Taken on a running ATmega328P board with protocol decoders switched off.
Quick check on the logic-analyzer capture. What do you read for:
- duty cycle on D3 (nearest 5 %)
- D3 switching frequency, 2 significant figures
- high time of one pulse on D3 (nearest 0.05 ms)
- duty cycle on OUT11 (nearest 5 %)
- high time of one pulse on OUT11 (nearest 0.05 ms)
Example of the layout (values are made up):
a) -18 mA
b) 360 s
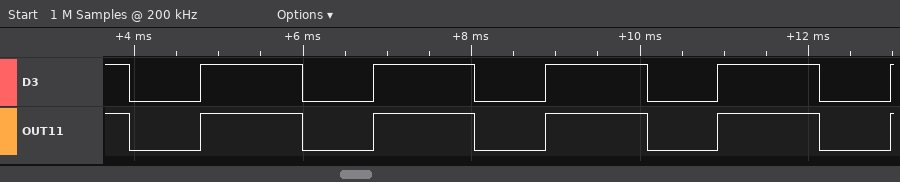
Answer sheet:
a) 60 %
b) 490 Hz
c) 1.20 ms
d) 60 %
e) 1.20 ms
